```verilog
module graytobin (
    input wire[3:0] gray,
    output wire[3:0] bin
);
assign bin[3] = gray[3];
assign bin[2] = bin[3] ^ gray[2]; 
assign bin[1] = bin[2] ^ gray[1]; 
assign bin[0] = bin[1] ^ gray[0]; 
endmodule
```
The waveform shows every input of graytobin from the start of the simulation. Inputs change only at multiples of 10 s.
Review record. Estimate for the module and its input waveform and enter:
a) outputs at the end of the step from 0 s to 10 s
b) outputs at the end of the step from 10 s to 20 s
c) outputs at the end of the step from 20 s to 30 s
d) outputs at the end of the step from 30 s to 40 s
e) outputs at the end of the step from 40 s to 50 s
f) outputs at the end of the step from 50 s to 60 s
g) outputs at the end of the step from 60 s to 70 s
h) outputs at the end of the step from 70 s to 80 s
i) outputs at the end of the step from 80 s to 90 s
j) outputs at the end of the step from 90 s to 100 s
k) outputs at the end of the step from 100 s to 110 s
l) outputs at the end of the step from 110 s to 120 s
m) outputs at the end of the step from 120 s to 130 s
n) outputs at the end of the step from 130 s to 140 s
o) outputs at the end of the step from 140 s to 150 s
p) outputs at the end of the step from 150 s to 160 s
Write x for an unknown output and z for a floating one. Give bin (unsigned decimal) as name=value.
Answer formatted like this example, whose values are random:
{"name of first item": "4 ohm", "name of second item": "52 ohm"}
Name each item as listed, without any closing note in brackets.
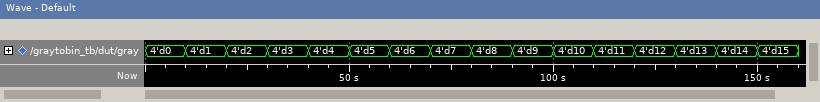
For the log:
{"outputs at the end of the step from 0 s to 10 s": "bin=0", "outputs at the end of the step from 10 s to 20 s": "bin=1", "outputs at the end of the step from 20 s to 30 s": "bin=3", "outputs at the end of the step from 30 s to 40 s": "bin=2", "outputs at the end of the step from 40 s to 50 s": "bin=7", "outputs at the end of the step from 50 s to 60 s": "bin=6", "outputs at the end of the step from 60 s to 70 s": "bin=4", "outputs at the end of the step from 70 s to 80 s": "bin=5", "outputs at the end of the step from 80 s to 90 s": "bin=15", "outputs at the end of the step from 90 s to 100 s": "bin=14", "outputs at the end of the step from 100 s to 110 s": "bin=12", "outputs at the end of the step from 110 s to 120 s": "bin=13", "outputs at the end of the step from 120 s to 130 s": "bin=8", "outputs at the end of the step from 130 s to 140 s": "bin=9", "outputs at the end of the step from 140 s to 150 s": "bin=11", "outputs at the end of the step from 150 s to 160 s": "bin=10"}
